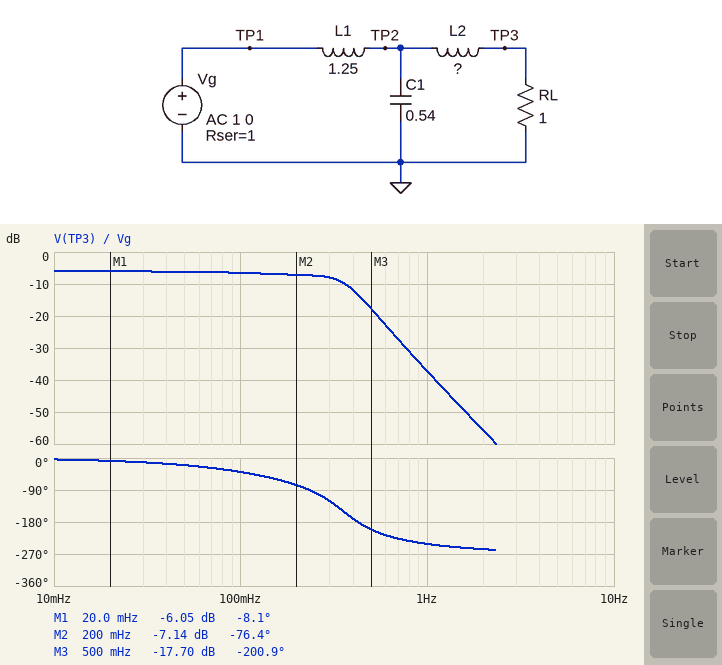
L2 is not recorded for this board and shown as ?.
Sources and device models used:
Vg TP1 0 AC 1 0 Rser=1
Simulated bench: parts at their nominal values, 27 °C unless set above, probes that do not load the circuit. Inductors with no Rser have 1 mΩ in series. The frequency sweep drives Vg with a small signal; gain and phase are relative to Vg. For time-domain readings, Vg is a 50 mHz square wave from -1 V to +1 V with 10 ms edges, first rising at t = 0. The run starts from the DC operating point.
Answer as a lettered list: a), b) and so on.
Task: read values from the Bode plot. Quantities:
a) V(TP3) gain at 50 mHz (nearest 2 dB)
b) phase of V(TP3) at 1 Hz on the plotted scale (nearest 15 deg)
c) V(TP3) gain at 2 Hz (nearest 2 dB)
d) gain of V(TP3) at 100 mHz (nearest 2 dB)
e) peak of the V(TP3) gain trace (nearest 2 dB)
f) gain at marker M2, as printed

a) -6 dB
b) -240 deg
c) -56 dB
d) -6 dB
e) -6 dB
f) -7.14 dB
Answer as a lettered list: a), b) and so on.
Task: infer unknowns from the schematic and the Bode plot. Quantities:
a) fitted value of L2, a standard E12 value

a) 470 mH
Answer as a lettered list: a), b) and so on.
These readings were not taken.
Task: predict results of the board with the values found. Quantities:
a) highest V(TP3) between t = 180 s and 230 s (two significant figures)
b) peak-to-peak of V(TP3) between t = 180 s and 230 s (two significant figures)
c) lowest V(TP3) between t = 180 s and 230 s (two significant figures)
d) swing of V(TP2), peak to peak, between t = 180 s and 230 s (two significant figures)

a) 530 mV
b) 1.1 V
c) -530 mV
d) 1.2 V
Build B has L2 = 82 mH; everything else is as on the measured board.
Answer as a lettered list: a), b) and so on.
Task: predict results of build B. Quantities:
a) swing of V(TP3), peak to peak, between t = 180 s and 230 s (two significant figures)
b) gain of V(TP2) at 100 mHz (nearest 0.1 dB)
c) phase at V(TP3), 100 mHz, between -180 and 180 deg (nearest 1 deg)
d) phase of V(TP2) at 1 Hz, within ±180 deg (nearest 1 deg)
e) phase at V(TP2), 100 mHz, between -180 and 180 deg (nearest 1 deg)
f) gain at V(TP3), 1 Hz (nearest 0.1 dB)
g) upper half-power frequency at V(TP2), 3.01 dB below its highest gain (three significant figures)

a) 1.0 V
b) -6.3 dB
c) -34 deg
d) -157 deg
e) -31 deg
f) -28.5 dB
g) 264 mHz
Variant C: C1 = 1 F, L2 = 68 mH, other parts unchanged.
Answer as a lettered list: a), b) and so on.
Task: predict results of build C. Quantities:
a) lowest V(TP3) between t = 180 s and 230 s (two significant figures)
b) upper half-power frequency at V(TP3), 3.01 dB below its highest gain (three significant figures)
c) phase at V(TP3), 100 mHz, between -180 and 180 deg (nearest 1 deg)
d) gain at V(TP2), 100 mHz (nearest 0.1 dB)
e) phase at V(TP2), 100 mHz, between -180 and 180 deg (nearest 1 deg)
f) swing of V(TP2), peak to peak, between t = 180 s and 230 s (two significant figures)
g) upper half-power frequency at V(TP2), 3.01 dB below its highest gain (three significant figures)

a) -540 mV
b) 206 mHz
c) -44 deg
d) -6.3 dB
e) -42 deg
f) 1.1 V
g) 207 mHz
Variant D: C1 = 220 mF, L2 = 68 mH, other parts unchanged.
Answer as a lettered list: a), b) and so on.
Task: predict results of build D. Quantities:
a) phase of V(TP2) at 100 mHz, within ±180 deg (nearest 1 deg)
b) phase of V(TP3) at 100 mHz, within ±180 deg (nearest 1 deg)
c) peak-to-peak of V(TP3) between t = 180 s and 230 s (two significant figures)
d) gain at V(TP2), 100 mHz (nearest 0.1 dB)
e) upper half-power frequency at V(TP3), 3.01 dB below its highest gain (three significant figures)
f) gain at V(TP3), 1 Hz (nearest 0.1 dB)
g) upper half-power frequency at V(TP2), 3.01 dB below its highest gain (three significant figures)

a) -25 deg
b) -27 deg
c) 1.0 V
d) -6.5 dB
e) 280 mHz
f) -20.6 dB
g) 284 mHz
